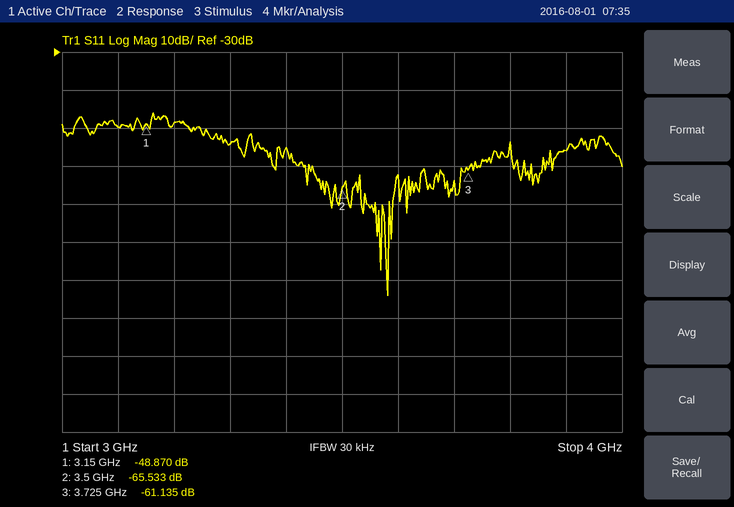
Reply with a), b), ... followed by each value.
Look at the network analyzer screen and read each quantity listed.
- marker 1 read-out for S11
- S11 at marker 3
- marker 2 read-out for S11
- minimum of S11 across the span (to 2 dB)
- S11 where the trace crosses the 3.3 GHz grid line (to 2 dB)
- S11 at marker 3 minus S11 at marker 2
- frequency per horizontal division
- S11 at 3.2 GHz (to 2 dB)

a) -48.870 dB
b) -61.135 dB
c) -65.533 dB
d) -94 dB
e) -54 dB
f) 4.398 dB
g) 100 MHz
h) -48 dB
